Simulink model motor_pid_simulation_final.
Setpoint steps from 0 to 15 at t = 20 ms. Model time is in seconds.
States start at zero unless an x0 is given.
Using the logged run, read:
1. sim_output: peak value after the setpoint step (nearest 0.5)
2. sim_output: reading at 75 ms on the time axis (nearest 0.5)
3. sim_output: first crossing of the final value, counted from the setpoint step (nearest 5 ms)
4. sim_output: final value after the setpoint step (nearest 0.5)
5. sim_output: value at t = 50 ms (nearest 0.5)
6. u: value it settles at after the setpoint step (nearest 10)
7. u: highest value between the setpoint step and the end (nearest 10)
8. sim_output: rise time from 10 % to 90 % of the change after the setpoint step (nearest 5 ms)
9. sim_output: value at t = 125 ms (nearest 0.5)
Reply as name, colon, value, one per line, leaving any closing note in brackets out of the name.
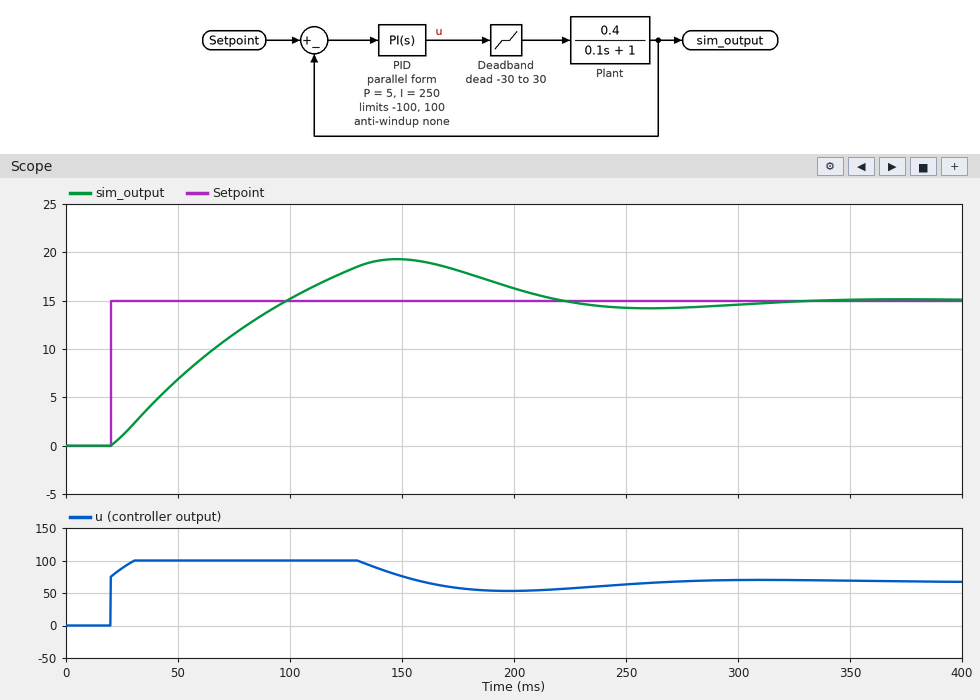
sim_output: peak value after the setpoint step: 19.5
sim_output: reading at 75 ms on the time axis: 11.5
sim_output: first crossing of the final value, counted from the setpoint step: 80 ms
sim_output: final value after the setpoint step: 15.0
sim_output: value at t = 50 ms: 7.0
u: value it settles at after the setpoint step: 70
u: highest value between the setpoint step and the end: 100
sim_output: rise time from 10 % to 90 % of the change after the setpoint step: 60 ms
sim_output: value at t = 125 ms: 18.0
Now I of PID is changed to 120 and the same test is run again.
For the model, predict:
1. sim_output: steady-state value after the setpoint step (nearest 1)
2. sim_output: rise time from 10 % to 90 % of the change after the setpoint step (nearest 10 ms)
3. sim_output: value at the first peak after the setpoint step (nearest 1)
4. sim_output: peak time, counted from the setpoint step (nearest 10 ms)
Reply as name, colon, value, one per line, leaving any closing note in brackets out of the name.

sim_output: steady-state value after the setpoint step: 15
sim_output: rise time from 10 % to 90 % of the change after the setpoint step: 80 ms
sim_output: value at the first peak after the setpoint step: 16
sim_output: peak time, counted from the setpoint step: 160 ms
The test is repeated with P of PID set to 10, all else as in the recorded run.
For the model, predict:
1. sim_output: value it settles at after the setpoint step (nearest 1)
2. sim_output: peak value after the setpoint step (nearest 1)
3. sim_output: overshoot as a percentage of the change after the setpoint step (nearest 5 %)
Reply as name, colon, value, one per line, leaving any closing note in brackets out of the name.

sim_output: value it settles at after the setpoint step: 15
sim_output: peak value after the setpoint step: 18
sim_output: overshoot as a percentage of the change after the setpoint step: 20 %
